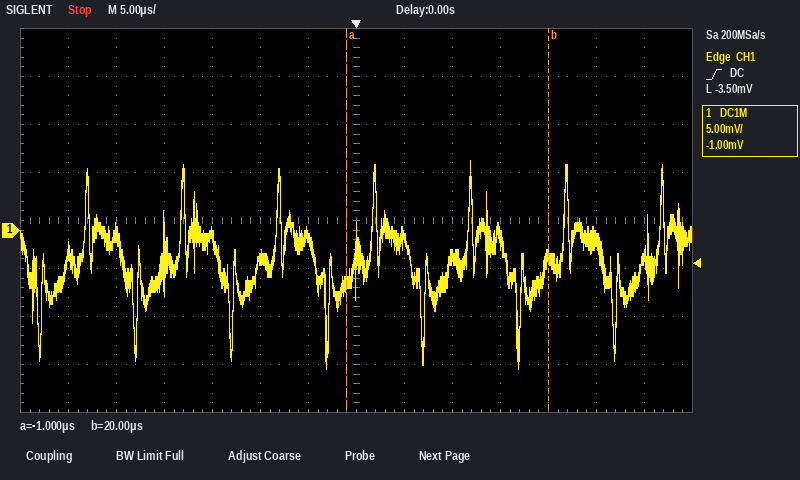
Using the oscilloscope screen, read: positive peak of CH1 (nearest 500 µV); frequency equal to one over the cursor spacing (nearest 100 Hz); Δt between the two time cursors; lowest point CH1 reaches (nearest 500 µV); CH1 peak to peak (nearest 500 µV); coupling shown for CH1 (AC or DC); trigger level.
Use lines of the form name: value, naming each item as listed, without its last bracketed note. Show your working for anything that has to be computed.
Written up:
positive peak of CH1: 7.0 mV
frequency equal to one over the cursor spacing: 1 / 21.0 µs ≈ 47.6 kHz
Δt between the two time cursors: 20 µs − (-1 µs) = 21.0 µs
lowest point CH1 reaches: -14.5 mV
CH1 peak to peak: 7.0 mV − (-14.5 mV) = 21.5 mV
coupling shown for CH1: DC
trigger level: -3.50 mV
